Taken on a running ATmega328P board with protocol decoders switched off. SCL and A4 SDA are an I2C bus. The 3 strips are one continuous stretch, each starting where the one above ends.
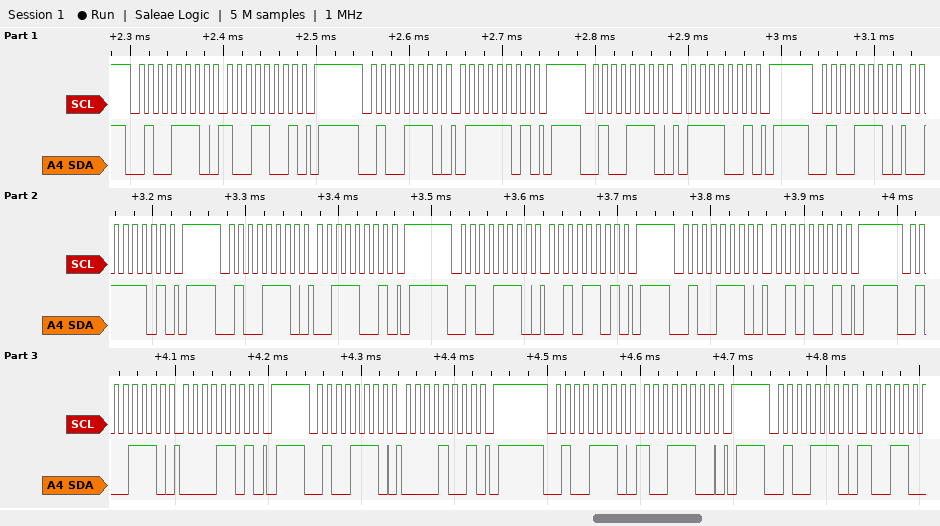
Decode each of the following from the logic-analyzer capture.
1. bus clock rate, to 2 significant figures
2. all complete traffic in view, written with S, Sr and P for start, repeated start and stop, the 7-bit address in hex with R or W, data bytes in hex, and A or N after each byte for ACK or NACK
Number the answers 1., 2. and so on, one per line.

1. 100 kHz
2. S 27W A 99 A P S 27W A 7D A P S 27W A 79 A P S 27W A 3D A P S 27W A 39 A P S 27W A 2D A P S 27W A 29 A P S 27W A 0D A P S 27W A 09 A P S 27W A 9C A P S 27W A
